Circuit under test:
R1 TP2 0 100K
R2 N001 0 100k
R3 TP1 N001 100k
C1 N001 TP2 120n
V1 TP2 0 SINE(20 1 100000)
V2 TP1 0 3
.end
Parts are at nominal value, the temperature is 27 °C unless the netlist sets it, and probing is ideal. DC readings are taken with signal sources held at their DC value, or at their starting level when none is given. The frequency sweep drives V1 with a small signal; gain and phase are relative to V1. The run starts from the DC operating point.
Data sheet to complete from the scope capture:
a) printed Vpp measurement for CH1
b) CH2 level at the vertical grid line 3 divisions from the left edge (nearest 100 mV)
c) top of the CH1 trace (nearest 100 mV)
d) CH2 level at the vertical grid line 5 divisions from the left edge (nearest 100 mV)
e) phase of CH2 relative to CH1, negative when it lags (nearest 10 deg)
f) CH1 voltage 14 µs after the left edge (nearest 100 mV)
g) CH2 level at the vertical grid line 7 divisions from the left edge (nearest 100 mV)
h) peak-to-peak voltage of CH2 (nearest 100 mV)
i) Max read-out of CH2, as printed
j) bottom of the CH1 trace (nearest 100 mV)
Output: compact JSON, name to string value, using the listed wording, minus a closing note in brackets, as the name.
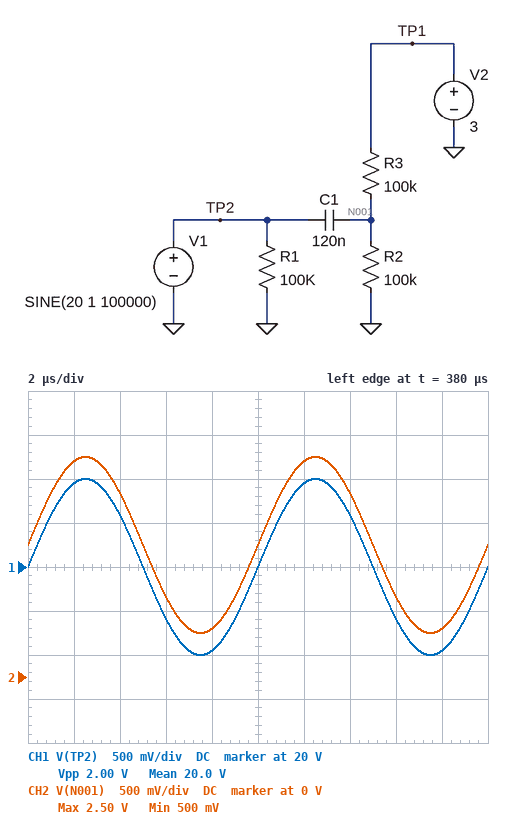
{"printed Vpp measurement for CH1": "2.00 V", "CH2 level at the vertical grid line 3 divisions from the left edge": "900 mV", "top of the CH1 trace": "21.0 V", "CH2 level at the vertical grid line 5 divisions from the left edge": "1.5 V", "phase of CH2 relative to CH1, negative when it lags": "0 deg", "CH1 voltage 14 µs after the left edge": "20.6 V", "CH2 level at the vertical grid line 7 divisions from the left edge": "2.1 V", "peak-to-peak voltage of CH2": "2.0 V", "Max read-out of CH2, as printed": "2.50 V", "bottom of the CH1 trace": "19.0 V"}
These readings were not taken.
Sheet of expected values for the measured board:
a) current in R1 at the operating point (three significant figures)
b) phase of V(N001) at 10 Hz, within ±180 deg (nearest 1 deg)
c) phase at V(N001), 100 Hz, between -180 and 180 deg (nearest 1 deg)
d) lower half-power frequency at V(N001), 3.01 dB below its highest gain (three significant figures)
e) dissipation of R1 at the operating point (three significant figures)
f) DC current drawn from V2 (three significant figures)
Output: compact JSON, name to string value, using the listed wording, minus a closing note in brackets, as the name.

{"current in R1 at the operating point": "200 µA", "phase of V(N001) at 10 Hz, within ±180 deg": "69 deg", "phase at V(N001), 100 Hz, between -180 and 180 deg": "15 deg", "lower half-power frequency at V(N001), 3.01 dB below its highest gain": "26.5 Hz", "dissipation of R1 at the operating point": "4.00 mW", "DC current drawn from V2": "15.0 µA"}
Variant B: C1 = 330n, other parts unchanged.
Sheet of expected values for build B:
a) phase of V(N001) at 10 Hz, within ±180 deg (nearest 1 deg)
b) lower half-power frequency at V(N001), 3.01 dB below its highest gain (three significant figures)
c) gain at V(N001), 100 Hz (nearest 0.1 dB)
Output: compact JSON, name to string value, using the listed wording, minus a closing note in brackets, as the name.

{"phase of V(N001) at 10 Hz, within ±180 deg": "44 deg", "lower half-power frequency at V(N001), 3.01 dB below its highest gain": "9.65 Hz", "gain at V(N001), 100 Hz": "0 dB"}
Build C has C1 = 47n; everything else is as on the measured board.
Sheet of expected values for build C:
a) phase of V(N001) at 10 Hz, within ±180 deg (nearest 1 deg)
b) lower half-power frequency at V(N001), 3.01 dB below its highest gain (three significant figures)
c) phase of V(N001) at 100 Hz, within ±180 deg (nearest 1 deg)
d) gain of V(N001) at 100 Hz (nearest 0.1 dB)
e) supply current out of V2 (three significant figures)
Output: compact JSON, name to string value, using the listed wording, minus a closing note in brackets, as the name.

{"phase of V(N001) at 10 Hz, within ±180 deg": "82 deg", "lower half-power frequency at V(N001), 3.01 dB below its highest gain": "67.7 Hz", "phase of V(N001) at 100 Hz, within ±180 deg": "34 deg", "gain of V(N001) at 100 Hz": "-1.6 dB", "supply current out of V2": "15.0 µA"}
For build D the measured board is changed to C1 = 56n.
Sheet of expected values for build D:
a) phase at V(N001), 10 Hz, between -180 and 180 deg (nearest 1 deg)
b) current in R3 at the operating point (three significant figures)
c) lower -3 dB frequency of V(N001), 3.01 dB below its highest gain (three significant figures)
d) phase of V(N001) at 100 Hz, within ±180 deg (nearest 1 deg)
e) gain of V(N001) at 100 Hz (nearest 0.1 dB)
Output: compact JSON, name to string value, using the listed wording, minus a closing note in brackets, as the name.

{"phase at V(N001), 10 Hz, between -180 and 180 deg": "80 deg", "current in R3 at the operating point": "15.0 µA", "lower -3 dB frequency of V(N001), 3.01 dB below its highest gain": "56.8 Hz", "phase of V(N001) at 100 Hz, within ±180 deg": "30 deg", "gain of V(N001) at 100 Hz": "-1.2 dB"}
